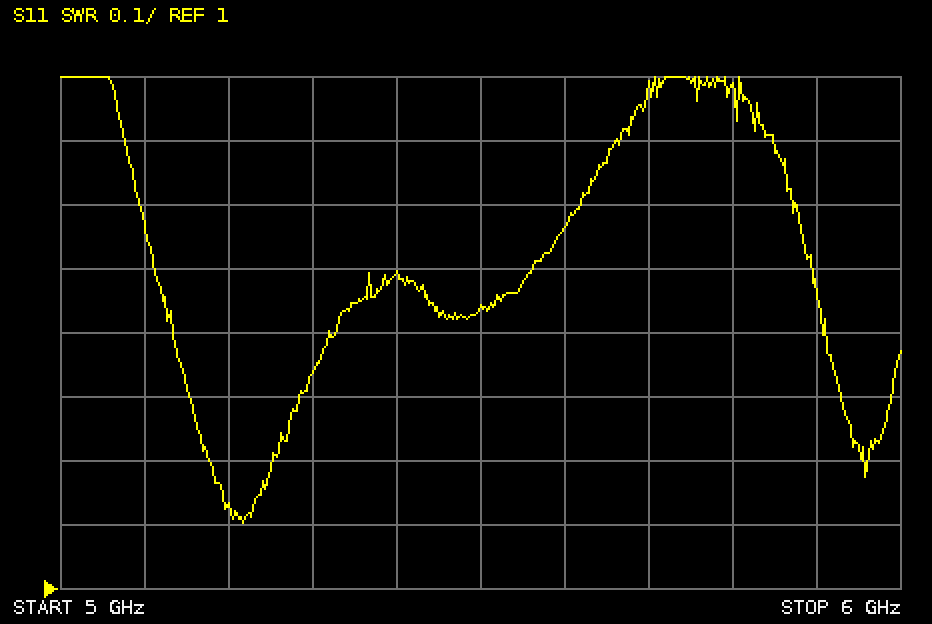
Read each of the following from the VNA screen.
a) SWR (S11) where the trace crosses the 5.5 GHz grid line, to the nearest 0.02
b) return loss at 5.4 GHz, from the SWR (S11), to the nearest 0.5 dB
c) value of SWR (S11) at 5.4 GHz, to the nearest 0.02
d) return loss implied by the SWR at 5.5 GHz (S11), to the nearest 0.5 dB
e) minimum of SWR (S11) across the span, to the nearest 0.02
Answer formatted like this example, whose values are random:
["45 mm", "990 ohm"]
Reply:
["1.44", "14.0 dB", "1.50", "15.0 dB", "1.10"]
